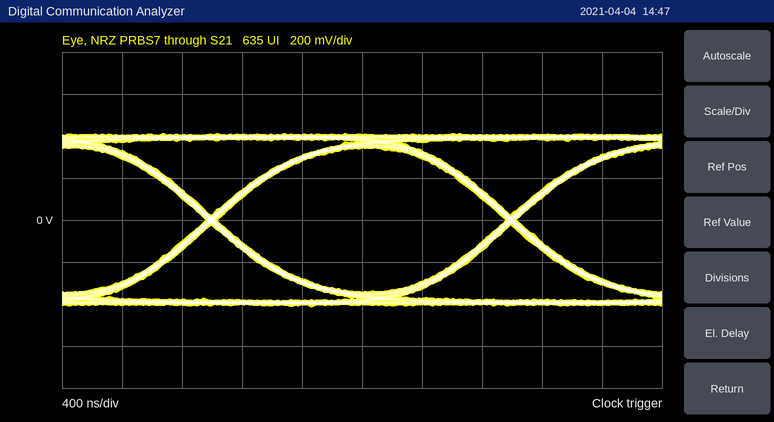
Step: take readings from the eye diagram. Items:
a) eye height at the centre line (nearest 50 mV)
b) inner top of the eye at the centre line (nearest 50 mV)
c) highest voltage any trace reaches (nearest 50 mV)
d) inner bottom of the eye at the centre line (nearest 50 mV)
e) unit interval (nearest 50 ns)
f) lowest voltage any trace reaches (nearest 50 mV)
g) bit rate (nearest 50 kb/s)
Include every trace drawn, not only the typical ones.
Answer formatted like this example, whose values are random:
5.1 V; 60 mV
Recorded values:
700 mV; 350 mV; 400 mV; -350 mV; 2.00 µs; -400 mV; 500 kb/s
